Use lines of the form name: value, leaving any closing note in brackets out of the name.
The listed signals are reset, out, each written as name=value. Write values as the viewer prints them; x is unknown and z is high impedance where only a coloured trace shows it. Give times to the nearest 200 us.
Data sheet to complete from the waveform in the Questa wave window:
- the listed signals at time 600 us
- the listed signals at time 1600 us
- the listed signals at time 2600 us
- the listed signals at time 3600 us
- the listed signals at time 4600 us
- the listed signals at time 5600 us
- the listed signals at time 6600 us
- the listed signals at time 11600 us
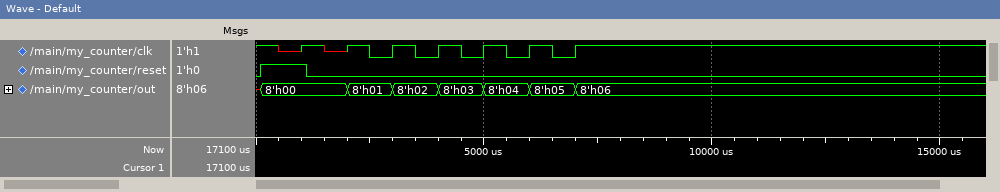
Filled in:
the listed signals at time 600 us: reset=1, out=8'h00
the listed signals at time 1600 us: reset=0, out=8'h00
the listed signals at time 2600 us: reset=0, out=8'h01
the listed signals at time 3600 us: reset=0, out=8'h02
the listed signals at time 4600 us: reset=0, out=8'h03
the listed signals at time 5600 us: reset=0, out=8'h04
the listed signals at time 6600 us: reset=0, out=8'h05
the listed signals at time 11600 us: reset=0, out=8'h06
